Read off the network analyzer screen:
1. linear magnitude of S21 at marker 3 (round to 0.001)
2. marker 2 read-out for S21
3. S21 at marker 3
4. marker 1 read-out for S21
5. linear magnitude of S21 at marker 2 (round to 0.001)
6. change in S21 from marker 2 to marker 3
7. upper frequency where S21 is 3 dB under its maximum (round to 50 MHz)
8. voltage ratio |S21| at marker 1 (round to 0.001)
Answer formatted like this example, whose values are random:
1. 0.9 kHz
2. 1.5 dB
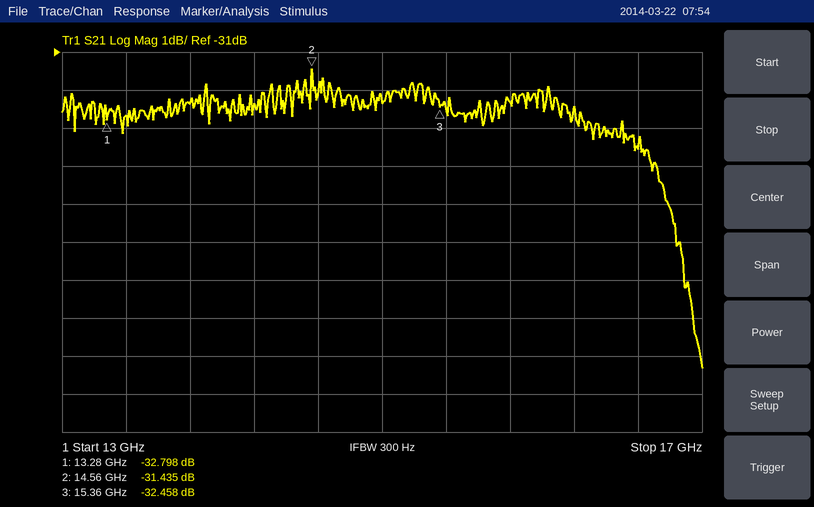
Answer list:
1. 0.024
2. -31.435 dB
3. -32.458 dB
4. -32.798 dB
5. 0.027
6. -1.023 dB
7. 16.75 GHz
8. 0.023
